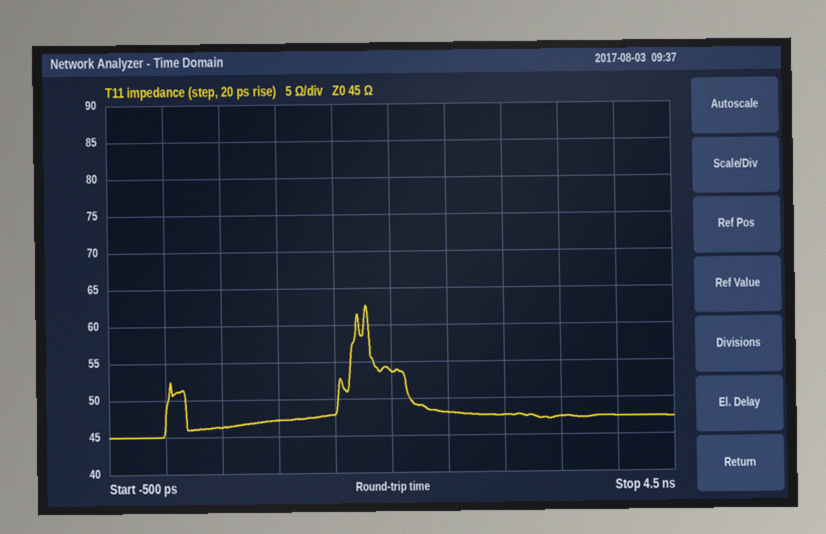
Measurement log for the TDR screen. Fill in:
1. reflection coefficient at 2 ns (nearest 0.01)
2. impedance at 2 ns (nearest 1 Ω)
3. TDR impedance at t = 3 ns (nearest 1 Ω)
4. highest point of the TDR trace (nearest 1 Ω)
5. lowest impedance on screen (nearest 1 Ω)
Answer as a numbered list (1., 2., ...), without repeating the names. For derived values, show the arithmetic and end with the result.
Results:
1. (54 − 45)/(54 + 45) ≈ +0.09
2. 54 Ω
3. 48 Ω
4. 63 Ω
5. 45 Ω
